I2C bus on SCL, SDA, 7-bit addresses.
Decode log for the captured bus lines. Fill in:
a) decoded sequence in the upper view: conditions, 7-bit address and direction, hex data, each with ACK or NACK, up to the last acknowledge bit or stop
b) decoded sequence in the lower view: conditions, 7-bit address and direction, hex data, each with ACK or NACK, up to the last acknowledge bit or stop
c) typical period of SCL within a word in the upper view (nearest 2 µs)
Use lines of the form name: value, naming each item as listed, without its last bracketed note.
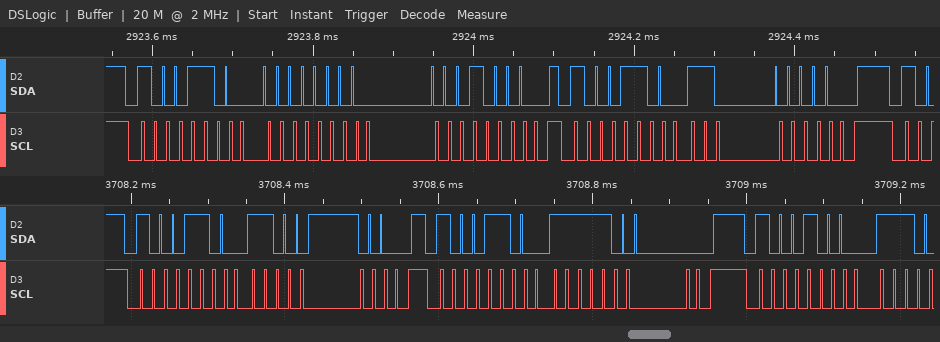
decoded sequence in the upper view: conditions, 7-bit address and direction, hex data, each with ACK or NACK, up to the last acknowledge bit or stop: start, address 46 write ACK, 00 ACK, 10 ACK, stop, start, address 46 write ACK, C0 ACK, stop
decoded sequence in the lower view: conditions, 7-bit address and direction, hex data, each with ACK or NACK, up to the last acknowledge bit or stop: start, address 46 write ACK, C0 ACK, stop, start, address 46 write ACK, F8 ACK, stop, start, address 44 write ACK
typical period of SCL within a word in the upper view: 16 µs
